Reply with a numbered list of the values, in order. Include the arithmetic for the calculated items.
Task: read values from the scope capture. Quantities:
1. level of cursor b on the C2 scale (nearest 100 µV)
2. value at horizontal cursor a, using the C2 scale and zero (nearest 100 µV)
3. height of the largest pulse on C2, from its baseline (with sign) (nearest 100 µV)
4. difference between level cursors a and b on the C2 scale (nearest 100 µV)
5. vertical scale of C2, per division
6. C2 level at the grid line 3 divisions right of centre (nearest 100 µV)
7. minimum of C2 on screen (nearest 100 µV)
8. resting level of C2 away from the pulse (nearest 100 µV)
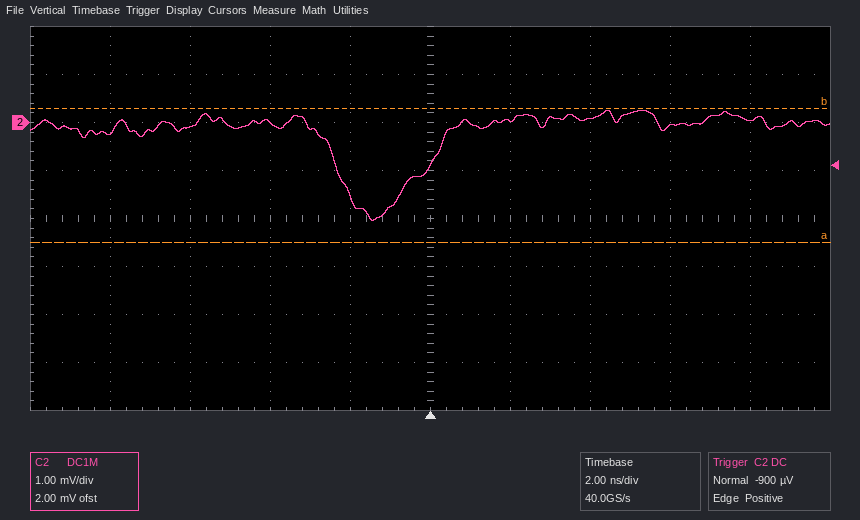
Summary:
1. 300 µV
2. -2.5 mV
3. -2.0 mV − (0.0 mV) = -2.0 mV
4. 2.8 mV
5. 1 mV
6. -100 µV
7. -2.0 mV
8. 0.0 mV
